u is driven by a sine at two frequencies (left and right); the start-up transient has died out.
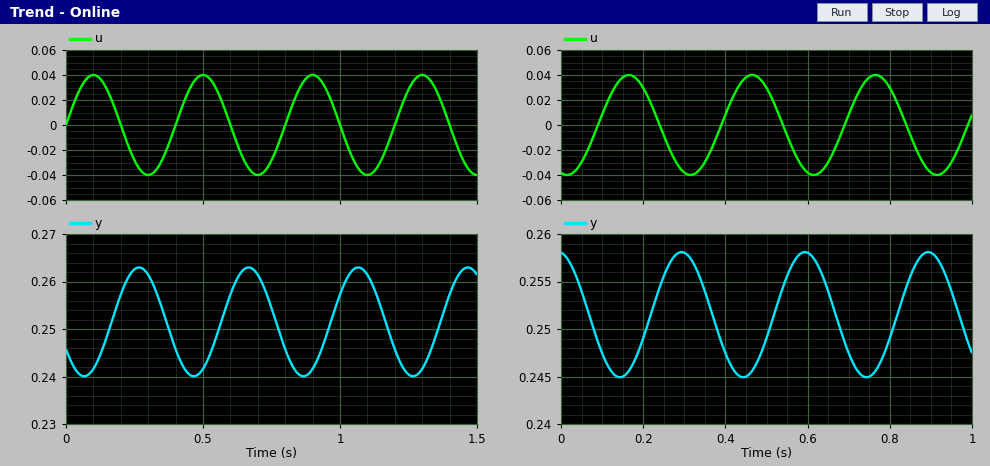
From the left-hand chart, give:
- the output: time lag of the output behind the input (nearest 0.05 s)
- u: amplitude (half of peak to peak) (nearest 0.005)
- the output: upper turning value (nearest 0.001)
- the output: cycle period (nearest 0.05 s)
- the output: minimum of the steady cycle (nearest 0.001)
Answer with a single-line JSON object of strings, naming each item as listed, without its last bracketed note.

{"the output: time lag of the output behind the input": "0.15 s", "u: amplitude (half of peak to peak)": "0.040", "the output: upper turning value": "0.263", "the output: cycle period": "0.40 s", "the output: minimum of the steady cycle": "0.240"}
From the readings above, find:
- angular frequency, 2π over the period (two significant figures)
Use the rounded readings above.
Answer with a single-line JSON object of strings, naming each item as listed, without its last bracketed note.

{"angular frequency, 2π over the period": "16 rad/s"}
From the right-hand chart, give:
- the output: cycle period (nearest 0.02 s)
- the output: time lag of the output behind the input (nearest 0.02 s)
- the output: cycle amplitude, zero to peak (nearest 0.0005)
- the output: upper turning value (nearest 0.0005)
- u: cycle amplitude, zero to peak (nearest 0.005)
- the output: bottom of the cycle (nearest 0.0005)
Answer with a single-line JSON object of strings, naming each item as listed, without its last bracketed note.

{"the output: cycle period": "0.30 s", "the output: time lag of the output behind the input": "0.12 s", "the output: cycle amplitude, zero to peak": "0.0065", "the output: upper turning value": "0.2580", "u: cycle amplitude, zero to peak": "0.040", "the output: bottom of the cycle": "0.2450"}
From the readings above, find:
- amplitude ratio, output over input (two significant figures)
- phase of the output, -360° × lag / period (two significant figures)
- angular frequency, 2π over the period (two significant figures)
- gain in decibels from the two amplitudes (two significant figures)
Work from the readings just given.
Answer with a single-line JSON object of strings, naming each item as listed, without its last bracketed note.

{"amplitude ratio, output over input": "0.16", "phase of the output, -360° × lag / period": "-140°", "angular frequency, 2π over the period": "21 rad/s", "gain in decibels from the two amplitudes": "-16 dB"}
